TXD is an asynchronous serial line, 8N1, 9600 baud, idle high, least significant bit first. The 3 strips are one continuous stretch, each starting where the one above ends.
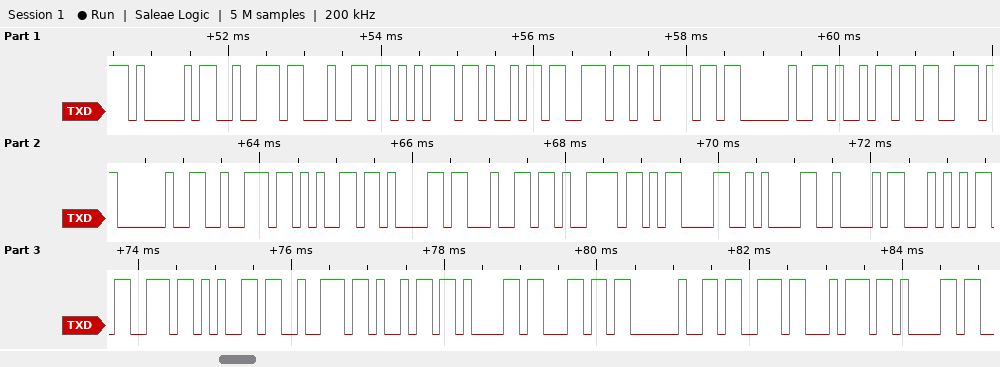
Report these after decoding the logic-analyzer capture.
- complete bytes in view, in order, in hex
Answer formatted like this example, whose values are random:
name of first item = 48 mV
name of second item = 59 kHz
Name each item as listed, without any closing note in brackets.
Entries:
complete bytes in view, in order, in hex = 41 72 64 75 69 6E 6F 20 69 73 20 72 65 61 64 79 0D 0A 42 54 73 65 72 69 61 6C 20 73 74 61
